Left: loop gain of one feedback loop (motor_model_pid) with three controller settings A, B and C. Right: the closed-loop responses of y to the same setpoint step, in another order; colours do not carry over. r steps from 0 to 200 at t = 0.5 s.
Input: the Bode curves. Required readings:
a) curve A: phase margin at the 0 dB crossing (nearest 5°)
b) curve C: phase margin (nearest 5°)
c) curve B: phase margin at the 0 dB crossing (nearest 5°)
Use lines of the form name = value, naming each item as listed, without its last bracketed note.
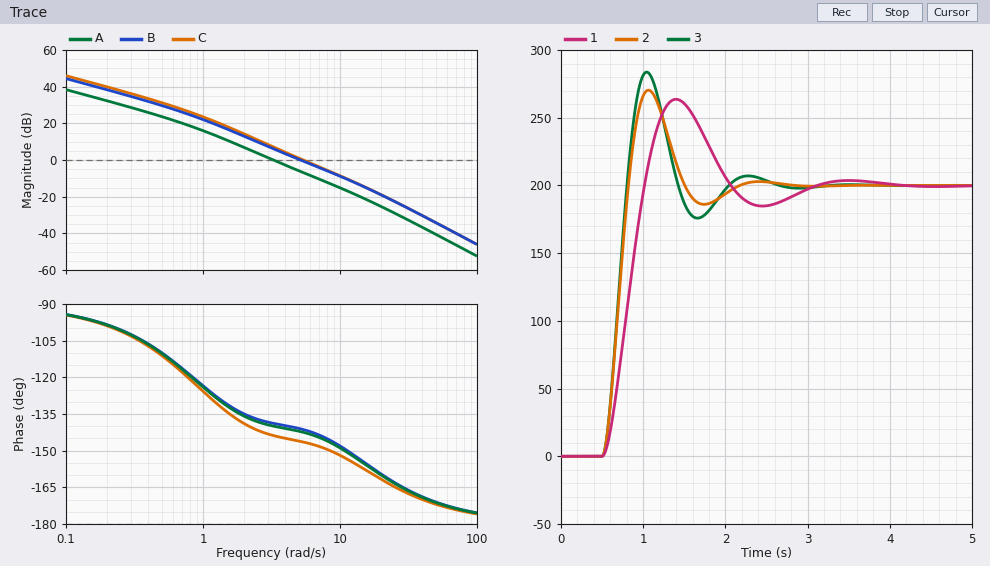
curve A: phase margin at the 0 dB crossing = 40°
curve C: phase margin = 35°
curve B: phase margin at the 0 dB crossing = 40°
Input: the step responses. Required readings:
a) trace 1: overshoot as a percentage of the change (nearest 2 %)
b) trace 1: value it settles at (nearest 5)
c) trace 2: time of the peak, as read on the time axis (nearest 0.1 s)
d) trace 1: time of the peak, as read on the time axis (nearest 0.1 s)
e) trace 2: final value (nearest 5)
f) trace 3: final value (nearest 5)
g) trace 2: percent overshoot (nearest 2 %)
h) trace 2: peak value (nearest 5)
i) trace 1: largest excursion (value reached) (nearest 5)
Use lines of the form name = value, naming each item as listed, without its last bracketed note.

trace 1: overshoot as a percentage of the change = 32 %
trace 1: value it settles at = 200
trace 2: time of the peak, as read on the time axis = 1.1 s
trace 1: time of the peak, as read on the time axis = 1.4 s
trace 2: final value = 200
trace 3: final value = 200
trace 2: percent overshoot = 36 %
trace 2: peak value = 270
trace 1: largest excursion (value reached) = 265
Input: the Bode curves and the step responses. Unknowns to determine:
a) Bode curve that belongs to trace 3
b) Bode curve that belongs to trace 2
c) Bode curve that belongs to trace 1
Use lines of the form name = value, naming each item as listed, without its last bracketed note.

Bode curve that belongs to trace 3 = C
Bode curve that belongs to trace 2 = B
Bode curve that belongs to trace 1 = A
